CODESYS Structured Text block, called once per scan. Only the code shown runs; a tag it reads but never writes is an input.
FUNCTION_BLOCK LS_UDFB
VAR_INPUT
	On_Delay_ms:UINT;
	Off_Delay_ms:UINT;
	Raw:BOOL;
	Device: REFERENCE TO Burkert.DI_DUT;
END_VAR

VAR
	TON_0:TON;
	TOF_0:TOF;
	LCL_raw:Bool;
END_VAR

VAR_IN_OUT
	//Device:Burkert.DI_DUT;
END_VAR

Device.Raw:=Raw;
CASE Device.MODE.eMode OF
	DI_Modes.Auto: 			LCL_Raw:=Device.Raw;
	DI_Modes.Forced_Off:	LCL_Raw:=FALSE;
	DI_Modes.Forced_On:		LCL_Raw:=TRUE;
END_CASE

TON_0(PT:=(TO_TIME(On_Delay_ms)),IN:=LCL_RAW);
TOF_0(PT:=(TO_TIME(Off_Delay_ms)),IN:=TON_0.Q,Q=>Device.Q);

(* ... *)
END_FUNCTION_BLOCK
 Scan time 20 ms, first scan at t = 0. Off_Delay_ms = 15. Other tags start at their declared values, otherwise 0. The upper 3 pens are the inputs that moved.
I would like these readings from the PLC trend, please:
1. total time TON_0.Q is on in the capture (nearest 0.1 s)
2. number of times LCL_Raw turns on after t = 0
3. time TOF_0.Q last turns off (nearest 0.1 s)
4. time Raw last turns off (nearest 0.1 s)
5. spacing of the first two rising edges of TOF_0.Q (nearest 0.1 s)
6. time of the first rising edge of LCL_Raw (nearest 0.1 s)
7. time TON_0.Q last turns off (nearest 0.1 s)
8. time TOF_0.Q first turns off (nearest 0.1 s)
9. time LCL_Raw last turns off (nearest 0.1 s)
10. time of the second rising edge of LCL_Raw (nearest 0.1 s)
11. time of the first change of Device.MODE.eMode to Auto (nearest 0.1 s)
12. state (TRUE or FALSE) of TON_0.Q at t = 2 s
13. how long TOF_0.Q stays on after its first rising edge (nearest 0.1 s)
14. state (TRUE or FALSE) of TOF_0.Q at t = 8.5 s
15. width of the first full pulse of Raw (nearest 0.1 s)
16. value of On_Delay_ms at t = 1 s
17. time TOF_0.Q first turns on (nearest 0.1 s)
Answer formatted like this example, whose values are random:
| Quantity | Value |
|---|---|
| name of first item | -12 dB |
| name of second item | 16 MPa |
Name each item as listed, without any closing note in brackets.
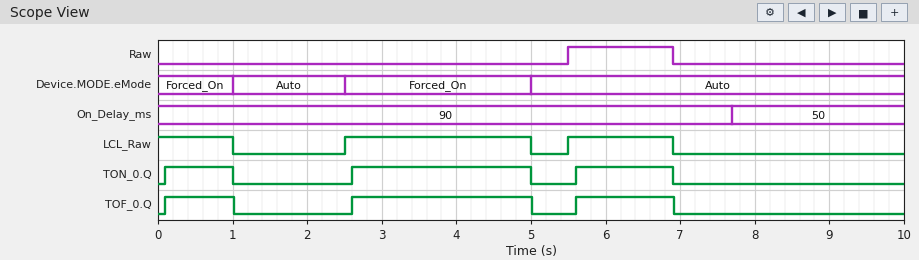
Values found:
| Quantity | Value |
|---|---|
| total time TON_0.Q is on in the capture | 4.6 s |
| number of times LCL_Raw turns on after t = 0 | 2 |
| time TOF_0.Q last turns off | 6.9 s |
| time Raw last turns off | 6.9 s |
| spacing of the first two rising edges of TOF_0.Q | 2.5 s |
| time of the first rising edge of LCL_Raw | 2.5 s |
| time TON_0.Q last turns off | 6.9 s |
| time TOF_0.Q first turns off | 1.0 s |
| time LCL_Raw last turns off | 6.9 s |
| time of the second rising edge of LCL_Raw | 5.5 s |
| time of the first change of Device.MODE.eMode to Auto | 1.0 s |
| state (TRUE or FALSE) of TON_0.Q at t = 2 s | FALSE |
| how long TOF_0.Q stays on after its first rising edge | 0.9 s |
| state (TRUE or FALSE) of TOF_0.Q at t = 8.5 s | FALSE |
| width of the first full pulse of Raw | 1.4 s |
| value of On_Delay_ms at t = 1 s | 90 |
| time TOF_0.Q first turns on | 0.1 s |
